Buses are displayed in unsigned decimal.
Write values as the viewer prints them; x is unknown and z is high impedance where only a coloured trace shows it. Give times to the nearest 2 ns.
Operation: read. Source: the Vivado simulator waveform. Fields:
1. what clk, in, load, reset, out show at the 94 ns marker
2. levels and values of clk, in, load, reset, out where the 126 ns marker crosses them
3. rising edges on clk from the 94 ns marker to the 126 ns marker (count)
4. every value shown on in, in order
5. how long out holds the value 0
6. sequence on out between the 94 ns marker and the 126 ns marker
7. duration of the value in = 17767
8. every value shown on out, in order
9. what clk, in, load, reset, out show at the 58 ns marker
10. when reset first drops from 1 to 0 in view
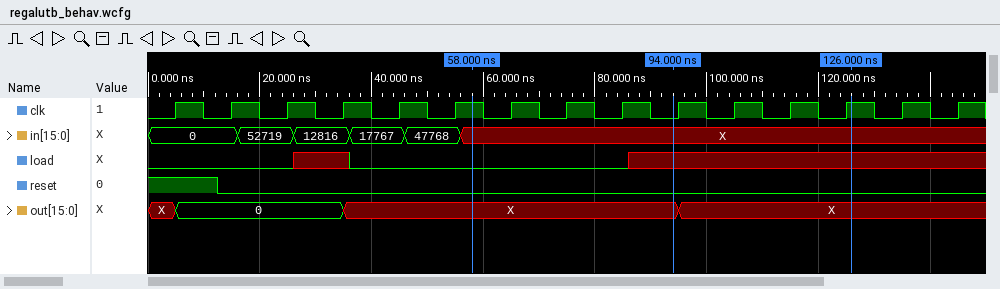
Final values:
clk=0, in=X, load=x, reset=0, out=X
clk=1, in=X, load=x, reset=0, out=X
4
0, 52719, 12816, 17767, 47768, X
30 ns
X, X
10 ns
X, 0, X, X
clk=1, in=X, load=0, reset=0, out=X
12 ns
